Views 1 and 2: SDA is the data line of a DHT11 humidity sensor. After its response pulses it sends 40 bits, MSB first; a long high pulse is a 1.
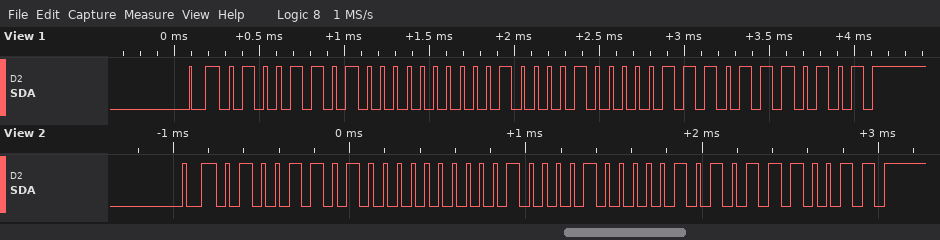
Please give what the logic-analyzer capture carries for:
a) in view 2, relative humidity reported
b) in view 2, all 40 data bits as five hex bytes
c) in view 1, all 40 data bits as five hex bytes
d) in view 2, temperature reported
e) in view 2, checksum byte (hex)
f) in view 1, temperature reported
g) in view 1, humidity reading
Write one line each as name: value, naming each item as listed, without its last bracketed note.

in view 2, relative humidity reported: 77 %
in view 2, all 40 data bits as five hex bytes: 4D 00 21 05 73
in view 1, all 40 data bits as five hex bytes: 4D 00 21 07 75
in view 2, temperature reported: 33.5 °C
in view 2, checksum byte: 0x73
in view 1, temperature reported: 33.7 °C
in view 1, humidity reading: 77 %
